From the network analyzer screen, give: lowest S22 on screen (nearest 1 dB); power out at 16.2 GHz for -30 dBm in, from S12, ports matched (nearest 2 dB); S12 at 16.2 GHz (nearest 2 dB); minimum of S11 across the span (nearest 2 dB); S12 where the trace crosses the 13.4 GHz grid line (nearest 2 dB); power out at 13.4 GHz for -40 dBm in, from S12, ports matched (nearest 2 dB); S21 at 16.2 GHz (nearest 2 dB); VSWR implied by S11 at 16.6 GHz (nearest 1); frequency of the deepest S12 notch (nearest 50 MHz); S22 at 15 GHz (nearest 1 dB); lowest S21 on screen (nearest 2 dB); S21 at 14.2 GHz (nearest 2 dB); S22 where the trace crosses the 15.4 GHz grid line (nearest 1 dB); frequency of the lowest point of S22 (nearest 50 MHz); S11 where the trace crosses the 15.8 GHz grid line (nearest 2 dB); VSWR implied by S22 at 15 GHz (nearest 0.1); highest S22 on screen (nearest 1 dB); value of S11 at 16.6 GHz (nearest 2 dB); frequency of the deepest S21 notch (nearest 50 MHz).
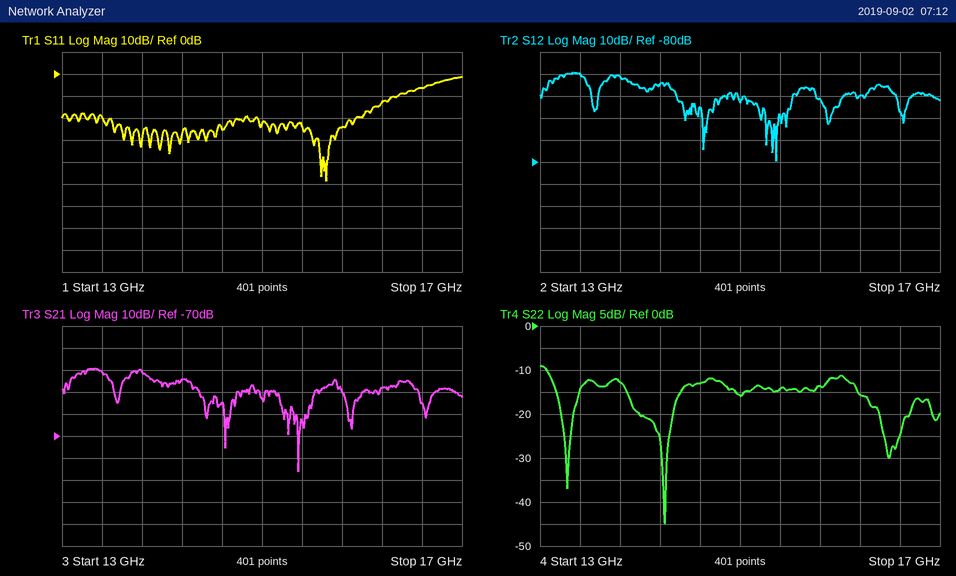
-45 dB
-80 dBm
-50 dB
-48 dB
-40 dB
-80 dBm
-48 dB
3
15.35 GHz
-16 dB
-86 dB
-44 dB
-14 dB
14.25 GHz
-24 dB
1.4
-9 dB
-6 dB
15.35 GHz
